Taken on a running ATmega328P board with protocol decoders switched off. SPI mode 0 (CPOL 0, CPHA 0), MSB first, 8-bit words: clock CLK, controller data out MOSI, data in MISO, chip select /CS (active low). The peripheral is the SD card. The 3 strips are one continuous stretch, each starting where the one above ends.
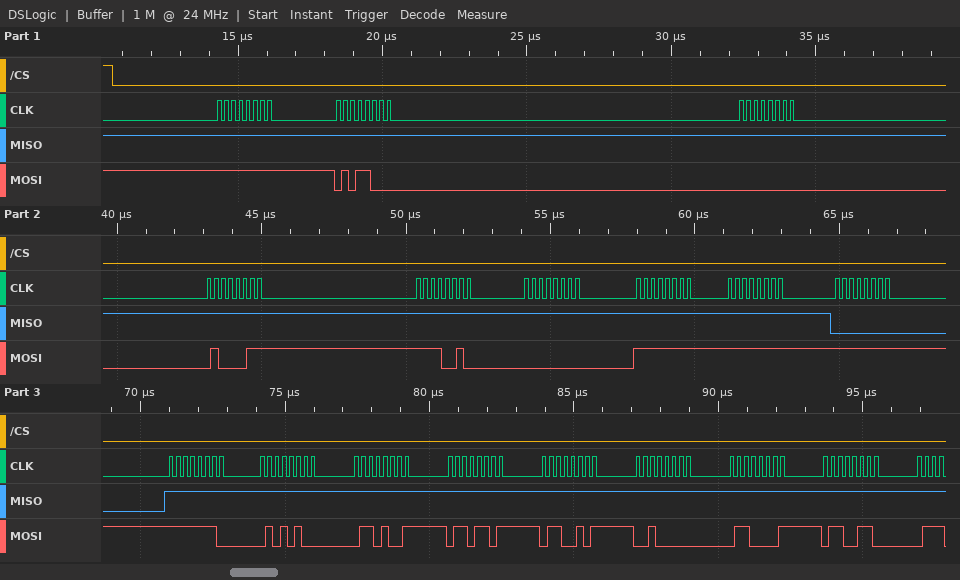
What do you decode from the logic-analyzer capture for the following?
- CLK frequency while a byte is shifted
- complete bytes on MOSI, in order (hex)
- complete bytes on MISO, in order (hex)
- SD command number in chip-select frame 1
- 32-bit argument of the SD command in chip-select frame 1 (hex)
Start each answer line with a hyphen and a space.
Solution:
- 4 MHz
- 0xFF 0x58 0x00 0x43 0xF2 0x00 0xFF 0xFF 0xFF 0xFE 0x54 0x69 0x6D 0x65 0x20 0x61 0x66
- 0xFF 0xFF 0xFF 0xFF 0xFF 0xFF 0xFF 0xFF 0x00 0xFF 0xFF 0xFF 0xFF 0xFF 0xFF 0xFF 0xFF
- CMD24
- 0x0043F200
